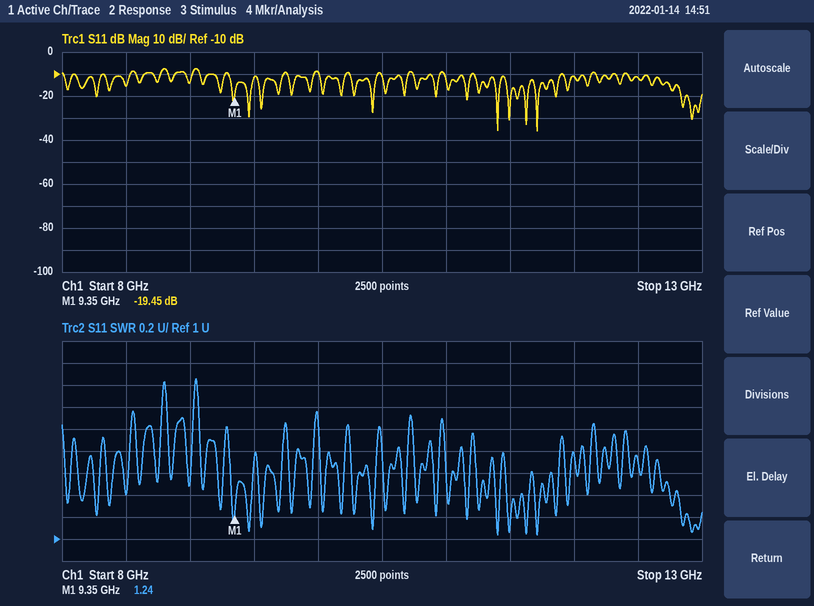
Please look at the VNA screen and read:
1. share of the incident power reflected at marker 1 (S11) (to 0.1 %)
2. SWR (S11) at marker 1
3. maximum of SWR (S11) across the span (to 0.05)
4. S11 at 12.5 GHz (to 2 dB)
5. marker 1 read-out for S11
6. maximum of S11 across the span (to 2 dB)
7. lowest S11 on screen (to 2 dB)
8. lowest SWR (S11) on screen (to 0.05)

1.1 %
1.24
2.45
-12 dB
-19.45 dB
-8 dB
-36 dB
1.05
